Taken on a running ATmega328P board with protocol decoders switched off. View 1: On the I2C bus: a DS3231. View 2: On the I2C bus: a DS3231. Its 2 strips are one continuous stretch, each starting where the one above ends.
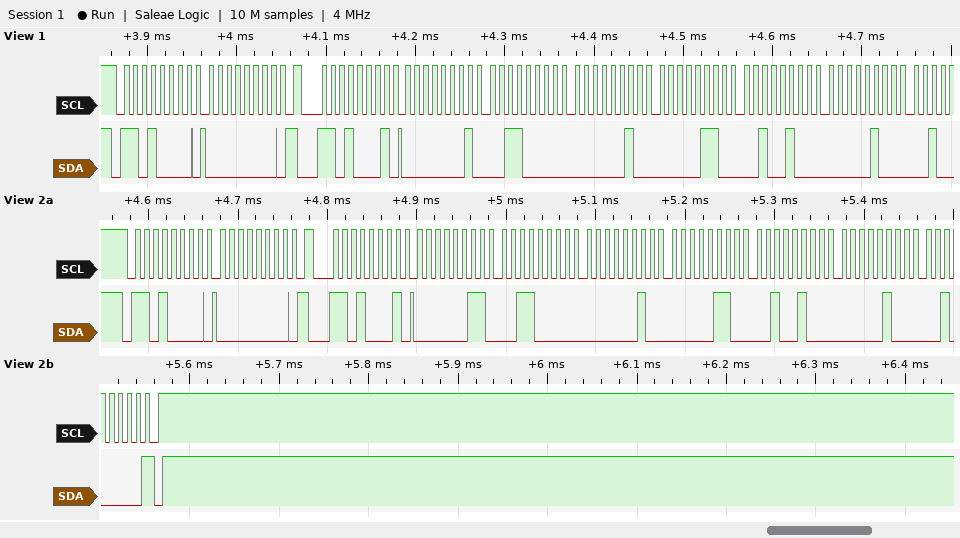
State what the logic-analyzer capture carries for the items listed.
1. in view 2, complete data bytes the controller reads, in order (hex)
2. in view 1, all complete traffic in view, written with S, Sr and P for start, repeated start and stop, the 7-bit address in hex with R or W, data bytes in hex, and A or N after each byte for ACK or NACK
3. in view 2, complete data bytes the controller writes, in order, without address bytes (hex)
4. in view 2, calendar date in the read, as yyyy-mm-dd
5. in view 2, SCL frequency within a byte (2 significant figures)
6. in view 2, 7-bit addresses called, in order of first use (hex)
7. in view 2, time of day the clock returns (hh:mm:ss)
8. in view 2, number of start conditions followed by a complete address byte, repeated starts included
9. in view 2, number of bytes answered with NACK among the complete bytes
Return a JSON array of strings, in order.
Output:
["03 30 02 06 24 04 20", "S 68W A 00 A Sr 68R A 01 A 30 A 02 A 06 A 24 A 04 A", "00", "2020-04-24", "100 kHz", "0x68", "02:30:03", "2", "1"]
